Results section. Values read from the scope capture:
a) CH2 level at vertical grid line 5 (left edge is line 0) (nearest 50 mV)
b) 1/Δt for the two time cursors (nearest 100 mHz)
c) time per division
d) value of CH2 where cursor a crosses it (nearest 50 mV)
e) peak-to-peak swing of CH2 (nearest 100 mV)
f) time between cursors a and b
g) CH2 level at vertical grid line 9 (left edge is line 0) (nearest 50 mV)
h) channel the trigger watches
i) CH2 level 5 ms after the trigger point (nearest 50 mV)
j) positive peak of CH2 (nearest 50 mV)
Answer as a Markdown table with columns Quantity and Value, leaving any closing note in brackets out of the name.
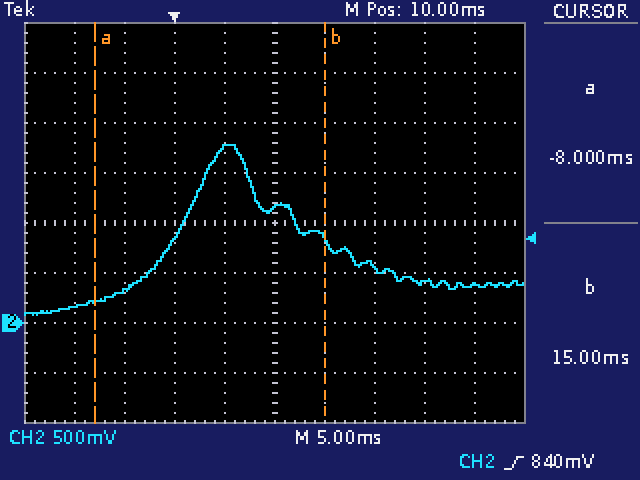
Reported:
| Quantity | Value |
|---|---|
| CH2 level at vertical grid line 5 (left edge is line 0) | 1.15 V |
| 1/Δt for the two time cursors | 43.5 Hz |
| time per division | 5 ms |
| value of CH2 where cursor a crosses it | 200 mV |
| peak-to-peak swing of CH2 | 1.70 V |
| time between cursors a and b | 23.0 ms |
| CH2 level at vertical grid line 9 (left edge is line 0) | 400 mV |
| channel the trigger watches | CH2 |
| CH2 level 5 ms after the trigger point | 1.75 V |
| positive peak of CH2 | 1.80 V |
